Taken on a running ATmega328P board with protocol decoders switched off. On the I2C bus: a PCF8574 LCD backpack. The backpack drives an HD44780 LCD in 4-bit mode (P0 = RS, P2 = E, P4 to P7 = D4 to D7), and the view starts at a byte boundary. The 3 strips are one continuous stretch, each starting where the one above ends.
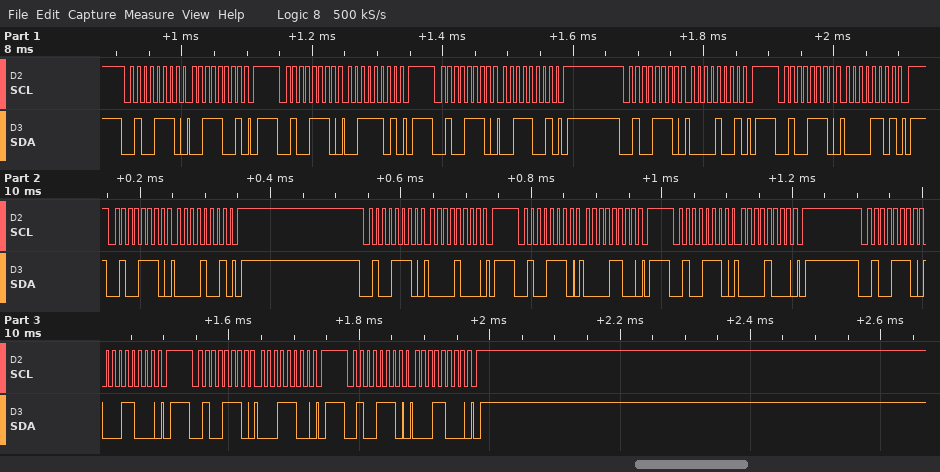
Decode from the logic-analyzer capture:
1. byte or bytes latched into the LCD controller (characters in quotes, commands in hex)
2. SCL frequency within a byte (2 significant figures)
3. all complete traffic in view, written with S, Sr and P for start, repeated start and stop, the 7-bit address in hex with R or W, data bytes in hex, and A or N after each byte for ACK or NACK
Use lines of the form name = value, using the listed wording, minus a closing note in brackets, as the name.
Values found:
byte or bytes latched into the LCD controller = '0' 0x01
SCL frequency within a byte = 100 kHz
all complete traffic in view, written with S, Sr and P for start, repeated start and stop, the 7-bit address in hex with R or W, data bytes in hex, and A or N after each byte for ACK or NACK = S 27W A 39 A P S 27W A 3D A P S 27W A 39 A P S 27W A 09 A P S 27W A 0D A P S 27W A 09 A P S 27W A 08 A P S 27W A 0C A P S 27W A 08 A P S 27W A 18 A P S 27W A 1C A P S 27W A 18 A P
